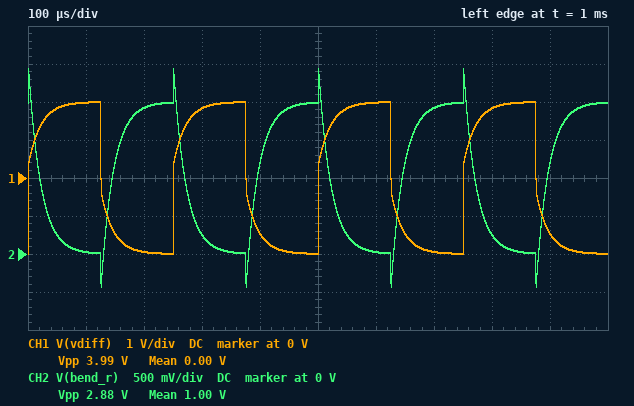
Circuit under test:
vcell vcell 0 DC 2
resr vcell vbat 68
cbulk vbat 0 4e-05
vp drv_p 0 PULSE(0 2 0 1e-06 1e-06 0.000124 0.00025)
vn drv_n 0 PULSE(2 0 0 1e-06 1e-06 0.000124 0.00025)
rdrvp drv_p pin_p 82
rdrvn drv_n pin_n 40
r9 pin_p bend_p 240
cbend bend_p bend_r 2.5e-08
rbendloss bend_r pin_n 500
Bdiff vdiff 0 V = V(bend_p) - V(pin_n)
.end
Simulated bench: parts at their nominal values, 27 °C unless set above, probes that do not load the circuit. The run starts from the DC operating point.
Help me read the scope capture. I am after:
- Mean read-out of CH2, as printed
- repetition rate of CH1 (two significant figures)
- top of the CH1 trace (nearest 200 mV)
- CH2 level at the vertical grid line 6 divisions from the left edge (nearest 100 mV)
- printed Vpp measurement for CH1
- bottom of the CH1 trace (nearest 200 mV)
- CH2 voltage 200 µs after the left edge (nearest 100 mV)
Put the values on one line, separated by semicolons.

1.00 V; 4.0 kHz; 2.0 V; 0 V; 3.99 V; -2.0 V; 1.9 V
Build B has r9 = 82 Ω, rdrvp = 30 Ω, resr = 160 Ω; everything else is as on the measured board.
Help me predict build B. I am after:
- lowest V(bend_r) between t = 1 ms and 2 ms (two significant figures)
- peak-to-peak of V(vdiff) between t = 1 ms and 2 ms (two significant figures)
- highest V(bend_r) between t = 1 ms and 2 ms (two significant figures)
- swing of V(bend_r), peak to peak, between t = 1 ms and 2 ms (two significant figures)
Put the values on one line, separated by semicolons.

-1.2 V; 4.0 V; 3.2 V; 4.4 V
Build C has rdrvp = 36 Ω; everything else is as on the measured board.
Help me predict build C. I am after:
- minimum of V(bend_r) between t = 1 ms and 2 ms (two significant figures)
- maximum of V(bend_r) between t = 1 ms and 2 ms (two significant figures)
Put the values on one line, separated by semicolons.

-580 mV; 2.6 V
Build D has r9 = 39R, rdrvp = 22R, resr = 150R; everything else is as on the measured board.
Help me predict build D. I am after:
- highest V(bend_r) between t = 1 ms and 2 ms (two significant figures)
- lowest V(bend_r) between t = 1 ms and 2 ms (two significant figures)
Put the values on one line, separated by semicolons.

3.5 V; -1.5 V
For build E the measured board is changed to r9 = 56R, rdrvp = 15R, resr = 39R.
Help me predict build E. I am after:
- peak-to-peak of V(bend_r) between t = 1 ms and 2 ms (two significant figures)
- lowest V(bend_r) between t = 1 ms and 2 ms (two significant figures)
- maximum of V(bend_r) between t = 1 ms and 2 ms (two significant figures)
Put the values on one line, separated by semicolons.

4.8 V; -1.4 V; 3.4 V
